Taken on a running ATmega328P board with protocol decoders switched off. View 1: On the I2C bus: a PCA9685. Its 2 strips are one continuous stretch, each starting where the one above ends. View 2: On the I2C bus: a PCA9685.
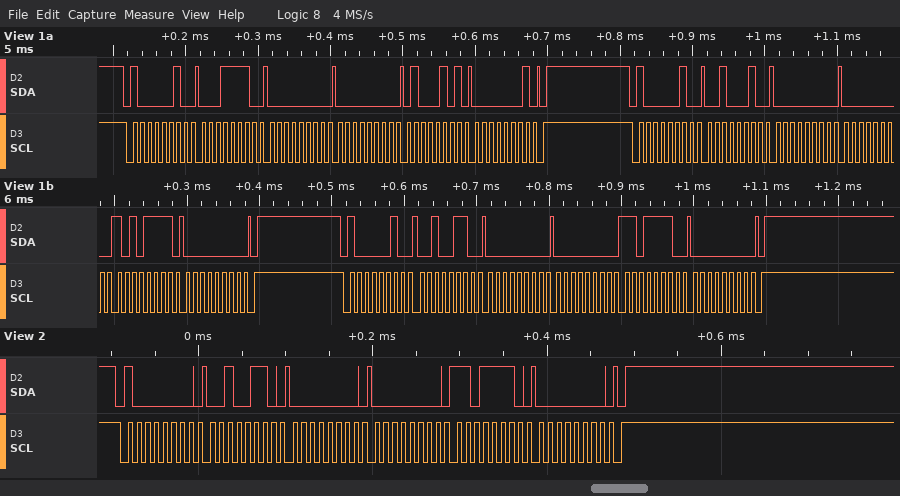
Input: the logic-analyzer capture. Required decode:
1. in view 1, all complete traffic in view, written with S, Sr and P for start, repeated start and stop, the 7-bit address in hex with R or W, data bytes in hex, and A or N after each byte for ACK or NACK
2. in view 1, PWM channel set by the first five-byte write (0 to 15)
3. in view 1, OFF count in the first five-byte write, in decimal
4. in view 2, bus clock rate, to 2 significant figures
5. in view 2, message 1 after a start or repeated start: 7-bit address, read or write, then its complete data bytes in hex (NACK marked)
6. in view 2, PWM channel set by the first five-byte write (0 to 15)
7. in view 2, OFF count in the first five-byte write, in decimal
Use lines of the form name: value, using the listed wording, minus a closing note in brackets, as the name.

in view 1, all complete traffic in view, written with S, Sr and P for start, repeated start and stop, the 7-bit address in hex with R or W, data bytes in hex, and A or N after each byte for ACK or NACK: S 41W A 1E A 00 A 00 A 45 A 01 A P S 41W A 22 A 00 A 00 A AF A 00 A P S 41W A 26 A 00 A 00 A DE A 00 A P
in view 1, PWM channel set by the first five-byte write: 6
in view 1, OFF count in the first five-byte write, in decimal: 325
in view 2, bus clock rate, to 2 significant figures: 100 kHz
in view 2, message 1 after a start or repeated start: 7-bit address, read or write, then its complete data bytes in hex: 0x40 write: 26 00 00 DE 00
in view 2, PWM channel set by the first five-byte write: 8
in view 2, OFF count in the first five-byte write, in decimal: 222
